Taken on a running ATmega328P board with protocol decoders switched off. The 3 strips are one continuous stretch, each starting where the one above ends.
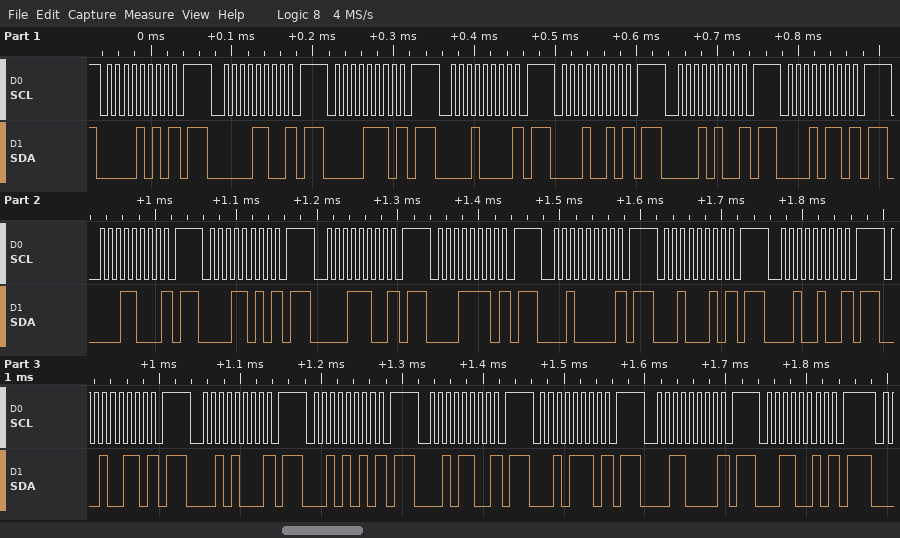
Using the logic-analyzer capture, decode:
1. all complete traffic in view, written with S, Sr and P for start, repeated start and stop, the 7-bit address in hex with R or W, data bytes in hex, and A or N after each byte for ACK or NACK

S 05W N P S 06W N P S 07W N P S 08W N P S 09W N P S 0AW N P S 0BW N P S 0CW N P S 0DW N P S 0EW N P S 0FW N P S 10W N P S 11W N P S 12W N P S 13W N P S 14W N P S 15W N P S 16W N P S 17W N P S 18W N P S 19W N P
